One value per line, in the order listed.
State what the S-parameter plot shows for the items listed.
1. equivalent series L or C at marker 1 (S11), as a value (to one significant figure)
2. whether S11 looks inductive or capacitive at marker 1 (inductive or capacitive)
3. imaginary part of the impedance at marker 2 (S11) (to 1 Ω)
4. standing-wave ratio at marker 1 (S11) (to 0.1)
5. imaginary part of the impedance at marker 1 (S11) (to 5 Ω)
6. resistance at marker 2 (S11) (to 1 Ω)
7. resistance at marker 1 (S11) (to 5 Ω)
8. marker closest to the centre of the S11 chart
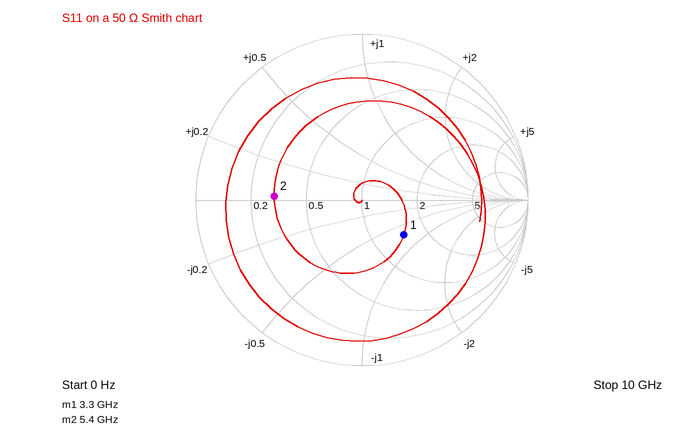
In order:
1 pF
capacitive
+1 Ω
2.0
-35 Ω
15 Ω
75 Ω
marker 1
